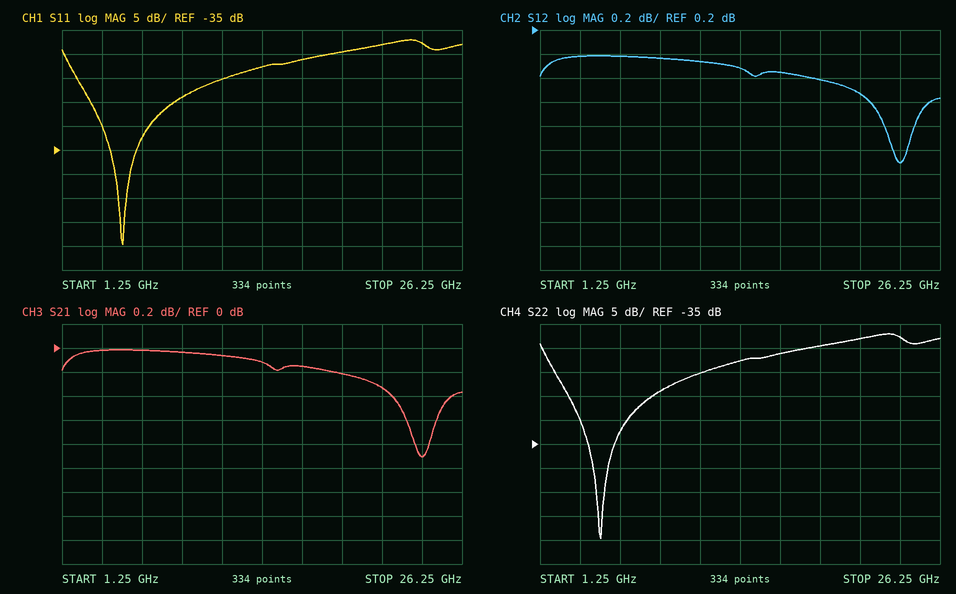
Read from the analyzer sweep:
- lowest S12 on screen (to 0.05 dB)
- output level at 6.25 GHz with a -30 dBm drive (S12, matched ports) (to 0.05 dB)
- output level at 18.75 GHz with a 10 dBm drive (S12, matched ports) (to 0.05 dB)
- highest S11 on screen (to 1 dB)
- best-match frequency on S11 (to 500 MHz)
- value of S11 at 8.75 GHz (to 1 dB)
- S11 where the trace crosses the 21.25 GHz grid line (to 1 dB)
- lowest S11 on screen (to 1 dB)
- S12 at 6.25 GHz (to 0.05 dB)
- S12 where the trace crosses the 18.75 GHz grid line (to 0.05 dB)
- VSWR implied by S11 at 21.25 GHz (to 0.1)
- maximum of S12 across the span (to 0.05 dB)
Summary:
-0.90 dB
-30.00 dBm
9.80 dBm
-12 dB
5.0 GHz
-24 dB
-13 dB
-55 dB
0.00 dB
-0.20 dB
1.6
0.00 dB
